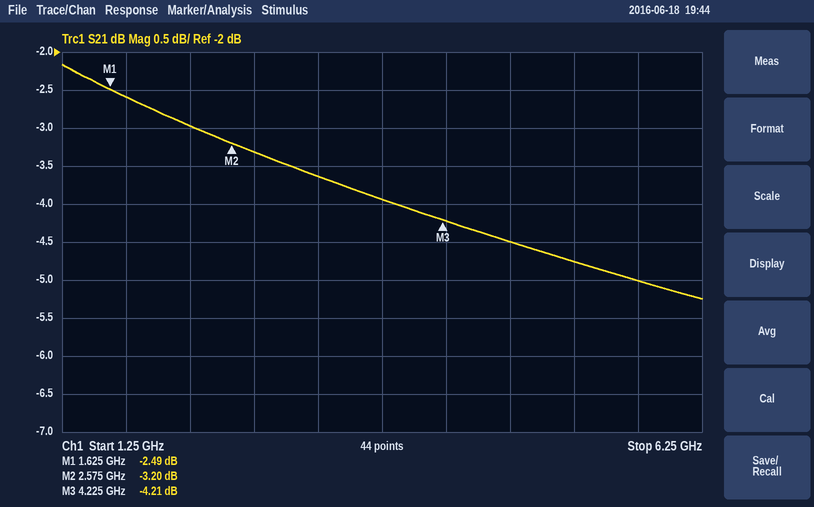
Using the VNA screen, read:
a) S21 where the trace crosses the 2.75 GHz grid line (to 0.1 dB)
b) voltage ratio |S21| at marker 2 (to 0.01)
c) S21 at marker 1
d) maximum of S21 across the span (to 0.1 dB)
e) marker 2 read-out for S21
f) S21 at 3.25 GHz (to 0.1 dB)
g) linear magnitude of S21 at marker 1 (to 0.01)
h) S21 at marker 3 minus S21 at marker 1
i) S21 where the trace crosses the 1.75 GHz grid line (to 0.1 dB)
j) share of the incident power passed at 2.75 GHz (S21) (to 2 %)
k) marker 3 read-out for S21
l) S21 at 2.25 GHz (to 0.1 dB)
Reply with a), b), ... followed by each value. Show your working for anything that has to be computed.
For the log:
a) -3.3 dB
b) 10^(-3.2/20) ≈ 0.69
c) -2.49 dB
d) -2.2 dB
e) -3.20 dB
f) -3.6 dB
g) 10^(-2.49/20) ≈ 0.75
h) -4.21 − (-2.49) = -1.72 dB
i) -2.6 dB
j) 10^(-3.3/10) ≈ 46.8 %, so 46 % to the nearest 2 %
k) -4.21 dB
l) -3.0 dB
